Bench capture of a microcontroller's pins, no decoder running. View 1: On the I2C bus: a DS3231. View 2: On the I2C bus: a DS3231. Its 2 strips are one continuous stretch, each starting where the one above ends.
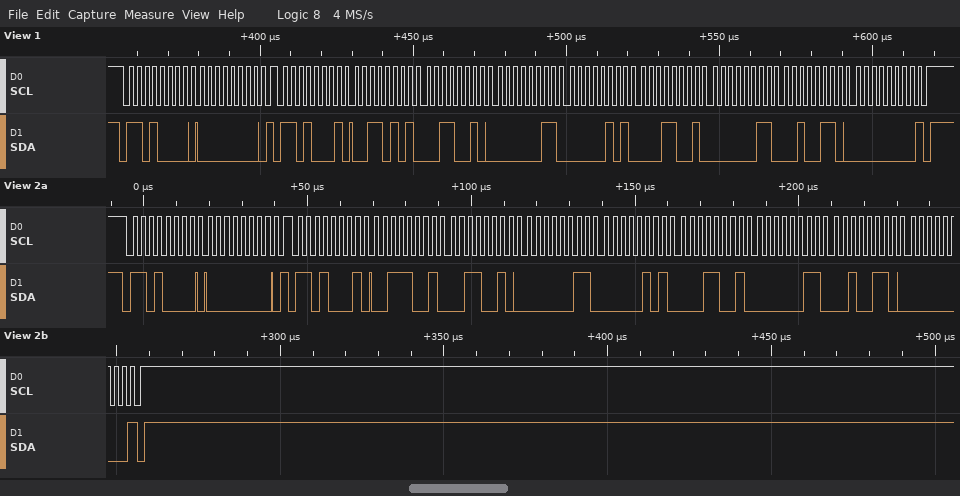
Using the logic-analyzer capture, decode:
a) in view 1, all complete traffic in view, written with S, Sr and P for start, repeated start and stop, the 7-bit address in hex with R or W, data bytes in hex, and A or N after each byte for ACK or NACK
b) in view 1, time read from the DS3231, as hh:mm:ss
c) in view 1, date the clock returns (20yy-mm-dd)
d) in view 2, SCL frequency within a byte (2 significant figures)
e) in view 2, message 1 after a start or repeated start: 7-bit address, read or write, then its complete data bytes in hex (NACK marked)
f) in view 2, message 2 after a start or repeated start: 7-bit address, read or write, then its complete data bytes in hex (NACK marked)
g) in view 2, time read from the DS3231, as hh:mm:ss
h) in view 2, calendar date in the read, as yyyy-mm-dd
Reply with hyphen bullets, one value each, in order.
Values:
- S 68W A 00 A Sr 68R A 35 A 32 A 03 A 05 A 19 A 03 A 26 A 00 N P
- 03:32:35
- 2026-03-19
- 400 kHz
- 0x68 write: 00
- 0x68 read: 39 32 03 05 19 03 26 00 NACK
- 03:32:39
- 2026-03-19
